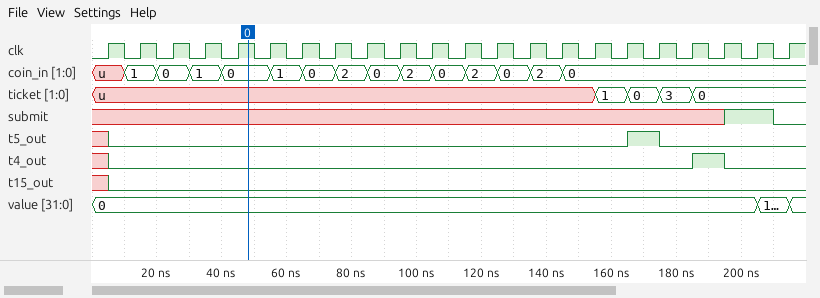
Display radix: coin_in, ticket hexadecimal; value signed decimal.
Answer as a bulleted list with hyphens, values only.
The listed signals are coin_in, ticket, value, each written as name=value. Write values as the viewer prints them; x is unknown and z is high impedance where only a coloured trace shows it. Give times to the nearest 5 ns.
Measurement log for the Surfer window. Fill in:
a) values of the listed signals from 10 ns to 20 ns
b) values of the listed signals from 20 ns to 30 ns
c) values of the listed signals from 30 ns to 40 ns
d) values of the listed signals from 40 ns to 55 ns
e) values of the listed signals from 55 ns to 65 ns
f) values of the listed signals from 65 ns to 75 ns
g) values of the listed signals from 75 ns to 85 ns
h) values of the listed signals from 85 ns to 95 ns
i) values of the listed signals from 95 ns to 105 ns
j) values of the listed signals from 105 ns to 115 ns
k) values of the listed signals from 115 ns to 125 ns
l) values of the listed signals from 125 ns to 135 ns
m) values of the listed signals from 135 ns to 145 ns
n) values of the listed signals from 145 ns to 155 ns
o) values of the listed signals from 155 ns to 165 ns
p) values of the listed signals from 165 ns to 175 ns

- coin_in=1, ticket=u, value=0
- coin_in=0, ticket=u, value=0
- coin_in=1, ticket=u, value=0
- coin_in=0, ticket=u, value=0
- coin_in=1, ticket=u, value=0
- coin_in=0, ticket=u, value=0
- coin_in=2, ticket=u, value=0
- coin_in=0, ticket=u, value=0
- coin_in=2, ticket=u, value=0
- coin_in=0, ticket=u, value=0
- coin_in=2, ticket=u, value=0
- coin_in=0, ticket=u, value=0
- coin_in=2, ticket=u, value=0
- coin_in=0, ticket=u, value=0
- coin_in=0, ticket=1, value=0
- coin_in=0, ticket=0, value=0
